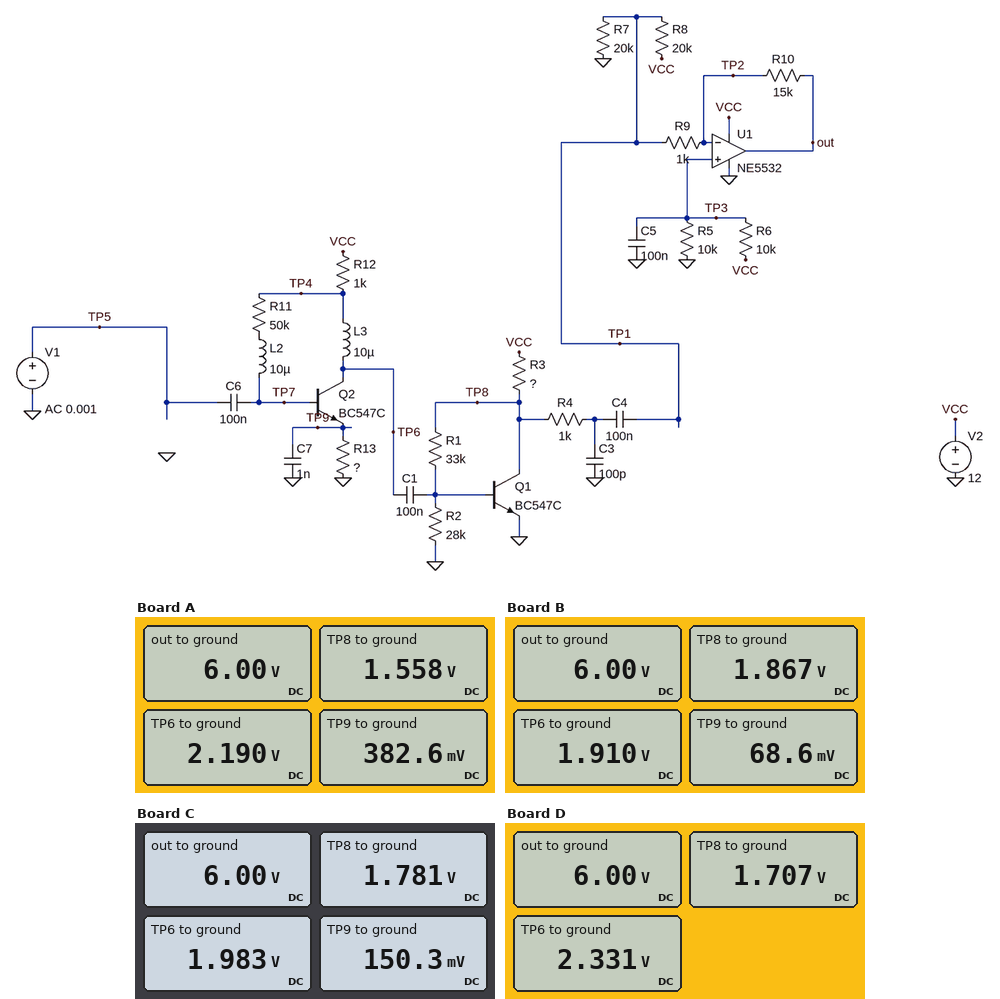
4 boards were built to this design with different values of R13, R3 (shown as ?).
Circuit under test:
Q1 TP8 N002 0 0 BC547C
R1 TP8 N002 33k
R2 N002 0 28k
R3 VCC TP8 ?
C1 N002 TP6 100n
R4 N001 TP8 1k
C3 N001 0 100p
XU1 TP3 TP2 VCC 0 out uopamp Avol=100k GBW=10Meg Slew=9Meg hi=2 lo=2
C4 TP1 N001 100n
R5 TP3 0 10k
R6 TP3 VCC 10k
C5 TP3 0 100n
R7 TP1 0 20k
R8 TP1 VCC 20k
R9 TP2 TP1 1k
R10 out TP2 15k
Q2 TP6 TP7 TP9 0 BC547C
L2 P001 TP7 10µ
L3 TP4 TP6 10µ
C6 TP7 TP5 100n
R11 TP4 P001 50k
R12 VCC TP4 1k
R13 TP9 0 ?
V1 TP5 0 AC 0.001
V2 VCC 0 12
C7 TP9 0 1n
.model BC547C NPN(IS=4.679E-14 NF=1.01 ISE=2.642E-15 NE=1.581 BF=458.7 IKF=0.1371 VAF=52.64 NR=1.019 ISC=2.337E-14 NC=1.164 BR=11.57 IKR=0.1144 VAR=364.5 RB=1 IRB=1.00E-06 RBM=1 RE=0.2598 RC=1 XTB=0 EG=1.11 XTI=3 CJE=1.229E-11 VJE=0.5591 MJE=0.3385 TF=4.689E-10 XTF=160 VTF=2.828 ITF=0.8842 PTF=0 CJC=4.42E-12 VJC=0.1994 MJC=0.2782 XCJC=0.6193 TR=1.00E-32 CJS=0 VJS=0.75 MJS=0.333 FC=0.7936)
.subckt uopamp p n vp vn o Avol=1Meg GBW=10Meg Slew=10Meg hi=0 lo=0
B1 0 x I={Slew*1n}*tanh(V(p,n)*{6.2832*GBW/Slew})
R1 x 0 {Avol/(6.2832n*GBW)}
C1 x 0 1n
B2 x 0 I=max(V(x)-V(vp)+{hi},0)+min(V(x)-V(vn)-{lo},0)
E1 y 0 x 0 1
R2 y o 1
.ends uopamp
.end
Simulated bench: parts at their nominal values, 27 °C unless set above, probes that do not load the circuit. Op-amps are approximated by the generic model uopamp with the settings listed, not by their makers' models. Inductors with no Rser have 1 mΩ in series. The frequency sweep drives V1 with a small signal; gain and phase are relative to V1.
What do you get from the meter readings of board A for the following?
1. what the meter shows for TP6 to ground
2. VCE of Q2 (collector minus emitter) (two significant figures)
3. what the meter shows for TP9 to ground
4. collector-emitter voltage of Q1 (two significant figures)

2.190 V
1.8 V
382.6 mV
1.6 V
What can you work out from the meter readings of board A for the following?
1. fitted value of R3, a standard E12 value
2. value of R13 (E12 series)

4.7 kΩ
39 Ω
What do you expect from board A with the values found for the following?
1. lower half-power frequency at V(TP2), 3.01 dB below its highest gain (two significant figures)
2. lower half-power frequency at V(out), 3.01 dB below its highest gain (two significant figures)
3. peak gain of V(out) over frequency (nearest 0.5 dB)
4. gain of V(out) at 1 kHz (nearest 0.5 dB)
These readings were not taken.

590 kHz
1.2 kHz
72.0 dB
66.5 dB
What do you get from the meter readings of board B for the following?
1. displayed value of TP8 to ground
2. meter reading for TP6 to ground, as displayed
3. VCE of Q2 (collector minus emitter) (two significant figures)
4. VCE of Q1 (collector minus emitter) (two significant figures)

1.867 V
1.910 V
1.8 V
1.9 V
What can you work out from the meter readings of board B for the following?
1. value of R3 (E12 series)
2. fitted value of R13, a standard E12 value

1.8 kΩ
6.8 Ω
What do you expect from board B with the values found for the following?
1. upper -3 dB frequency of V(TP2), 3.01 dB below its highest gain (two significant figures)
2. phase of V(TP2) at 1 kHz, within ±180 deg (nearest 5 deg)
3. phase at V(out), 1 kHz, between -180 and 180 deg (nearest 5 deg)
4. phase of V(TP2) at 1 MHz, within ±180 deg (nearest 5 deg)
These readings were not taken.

2.1 MHz
-85 deg
10 deg
-5 deg
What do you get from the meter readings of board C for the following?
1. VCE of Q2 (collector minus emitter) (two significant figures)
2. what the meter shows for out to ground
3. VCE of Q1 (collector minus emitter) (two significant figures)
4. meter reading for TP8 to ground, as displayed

1.8 V
6.00 V
1.8 V
1.781 V
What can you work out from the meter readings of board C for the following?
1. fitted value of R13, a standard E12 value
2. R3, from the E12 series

15 Ω
2.2 kΩ
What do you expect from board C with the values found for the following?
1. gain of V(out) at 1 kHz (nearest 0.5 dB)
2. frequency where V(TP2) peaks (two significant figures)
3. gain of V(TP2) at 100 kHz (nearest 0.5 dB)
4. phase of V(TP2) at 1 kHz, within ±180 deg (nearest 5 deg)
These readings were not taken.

70.0 dB
1.2 MHz
40.0 dB
-105 deg
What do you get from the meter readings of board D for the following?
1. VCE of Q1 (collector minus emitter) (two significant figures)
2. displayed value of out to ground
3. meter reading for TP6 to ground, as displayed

1.7 V
6.00 V
2.331 V
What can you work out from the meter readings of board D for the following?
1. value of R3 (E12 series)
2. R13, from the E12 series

2.7 kΩ
56 Ω
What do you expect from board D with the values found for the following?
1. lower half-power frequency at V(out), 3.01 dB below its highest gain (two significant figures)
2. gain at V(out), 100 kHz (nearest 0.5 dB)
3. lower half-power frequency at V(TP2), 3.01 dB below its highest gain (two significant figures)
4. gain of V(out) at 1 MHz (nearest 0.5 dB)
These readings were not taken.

1.3 kHz
69.5 dB
610 kHz
67.0 dB
